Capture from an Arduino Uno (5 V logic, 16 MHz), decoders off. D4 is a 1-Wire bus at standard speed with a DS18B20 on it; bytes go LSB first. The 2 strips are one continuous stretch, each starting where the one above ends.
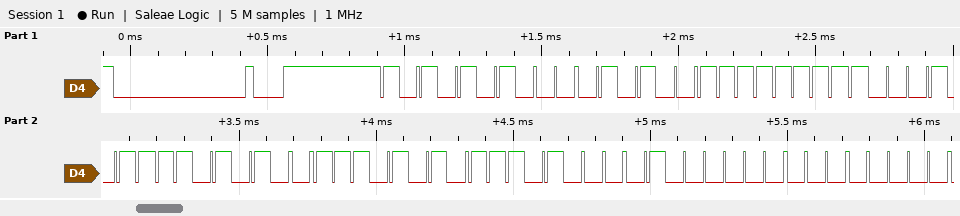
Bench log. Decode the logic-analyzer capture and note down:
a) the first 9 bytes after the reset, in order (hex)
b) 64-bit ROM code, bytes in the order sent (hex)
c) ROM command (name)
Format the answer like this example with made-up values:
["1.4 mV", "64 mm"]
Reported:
["55 28 FF D1 2B 57 17 02 00", "28 FF D1 2B 57 17 02 00", "Match ROM"]
